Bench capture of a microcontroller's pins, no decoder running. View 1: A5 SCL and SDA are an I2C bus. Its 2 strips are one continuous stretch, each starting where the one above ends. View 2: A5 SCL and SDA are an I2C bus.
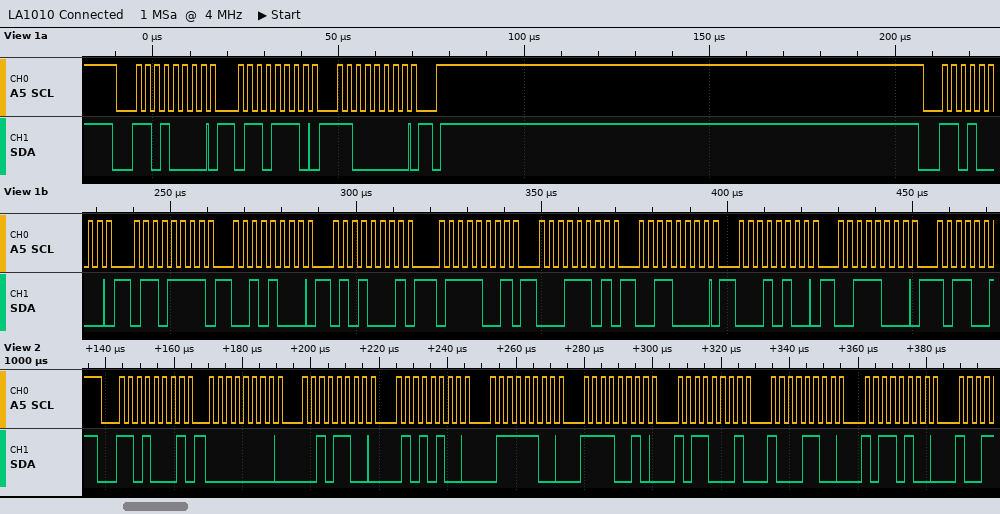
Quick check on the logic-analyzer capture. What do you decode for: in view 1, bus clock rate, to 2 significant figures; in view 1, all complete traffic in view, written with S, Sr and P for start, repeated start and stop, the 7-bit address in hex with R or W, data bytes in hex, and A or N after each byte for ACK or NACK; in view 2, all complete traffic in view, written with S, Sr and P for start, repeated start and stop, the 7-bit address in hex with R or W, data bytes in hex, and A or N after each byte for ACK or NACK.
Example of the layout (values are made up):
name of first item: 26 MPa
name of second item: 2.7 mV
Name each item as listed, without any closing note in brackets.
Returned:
in view 1, bus clock rate, to 2 significant figures: 400 kHz
in view 1, all complete traffic in view, written with S, Sr and P for start, repeated start and stop, the 7-bit address in hex with R or W, data bytes in hex, and A or N after each byte for ACK or NACK: S 68W A 6E A C0 A P S 68W A 6F A 28 A 51 A 79 A 1D A 30 A 14 A 38 A
in view 2, all complete traffic in view, written with S, Sr and P for start, repeated start and stop, the 7-bit address in hex with R or W, data bytes in hex, and A or N after each byte for ACK or NACK: S 68R A 00 A 2C A 54 A 7C A F2 A B1 A 8C A B4 A
